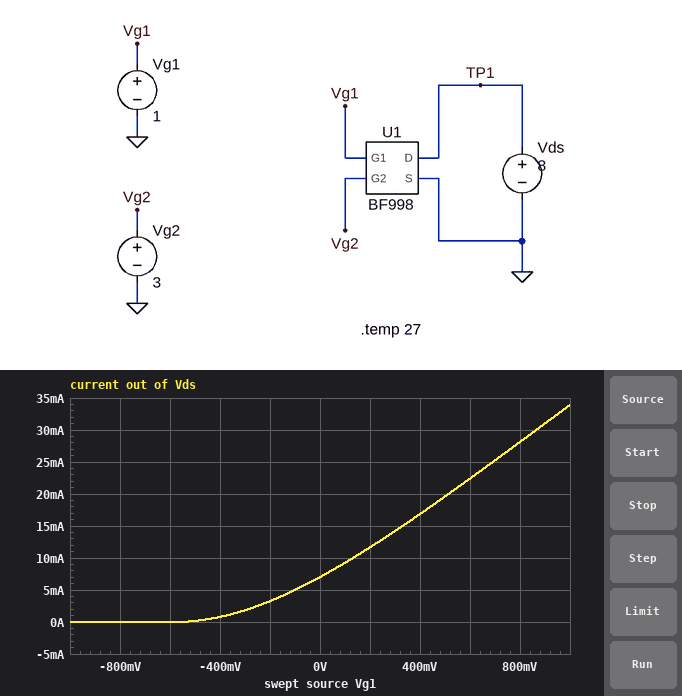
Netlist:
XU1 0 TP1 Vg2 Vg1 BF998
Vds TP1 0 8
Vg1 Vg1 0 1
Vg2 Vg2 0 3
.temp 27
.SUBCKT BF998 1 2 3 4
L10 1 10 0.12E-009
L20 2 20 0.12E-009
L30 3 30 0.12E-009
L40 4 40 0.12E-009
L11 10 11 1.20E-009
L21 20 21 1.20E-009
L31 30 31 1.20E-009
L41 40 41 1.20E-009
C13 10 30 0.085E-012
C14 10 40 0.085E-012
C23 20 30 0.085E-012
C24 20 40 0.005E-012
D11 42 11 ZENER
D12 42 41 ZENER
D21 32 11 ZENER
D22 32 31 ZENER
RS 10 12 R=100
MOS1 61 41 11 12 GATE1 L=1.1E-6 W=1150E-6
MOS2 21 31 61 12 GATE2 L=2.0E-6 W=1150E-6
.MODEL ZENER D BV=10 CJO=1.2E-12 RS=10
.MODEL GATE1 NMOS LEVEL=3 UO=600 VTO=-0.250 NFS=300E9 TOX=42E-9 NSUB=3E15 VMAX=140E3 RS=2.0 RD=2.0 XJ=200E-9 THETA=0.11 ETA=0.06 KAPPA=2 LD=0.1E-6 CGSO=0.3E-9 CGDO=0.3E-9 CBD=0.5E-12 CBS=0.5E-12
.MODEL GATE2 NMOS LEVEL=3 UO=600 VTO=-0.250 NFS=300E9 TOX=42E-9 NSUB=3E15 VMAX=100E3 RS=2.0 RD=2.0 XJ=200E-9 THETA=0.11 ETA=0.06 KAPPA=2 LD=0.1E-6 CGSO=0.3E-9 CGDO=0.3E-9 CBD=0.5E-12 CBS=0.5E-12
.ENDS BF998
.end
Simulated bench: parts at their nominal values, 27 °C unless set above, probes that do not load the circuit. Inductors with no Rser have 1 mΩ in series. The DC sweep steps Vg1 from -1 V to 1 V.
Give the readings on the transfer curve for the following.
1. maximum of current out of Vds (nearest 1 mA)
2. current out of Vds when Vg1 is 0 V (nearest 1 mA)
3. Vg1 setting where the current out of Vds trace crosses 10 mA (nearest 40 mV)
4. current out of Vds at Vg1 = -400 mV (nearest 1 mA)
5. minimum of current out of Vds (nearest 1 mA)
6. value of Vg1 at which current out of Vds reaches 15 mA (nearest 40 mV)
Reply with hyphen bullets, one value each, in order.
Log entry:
- 34 mA
- 7 mA
- 120 mV
- 1 mA
- 0 A
- 320 mV
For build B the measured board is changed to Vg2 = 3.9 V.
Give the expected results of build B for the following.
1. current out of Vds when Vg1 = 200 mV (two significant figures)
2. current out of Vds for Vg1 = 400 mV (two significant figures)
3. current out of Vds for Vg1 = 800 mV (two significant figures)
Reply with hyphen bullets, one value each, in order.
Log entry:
- 14 mA
- 20 mA
- 32 mA
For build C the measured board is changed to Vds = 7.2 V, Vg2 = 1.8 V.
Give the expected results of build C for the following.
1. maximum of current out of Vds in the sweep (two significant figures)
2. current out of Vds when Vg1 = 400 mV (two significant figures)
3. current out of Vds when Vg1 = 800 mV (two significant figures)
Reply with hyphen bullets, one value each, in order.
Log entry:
- 26 mA
- 13 mA
- 23 mA
